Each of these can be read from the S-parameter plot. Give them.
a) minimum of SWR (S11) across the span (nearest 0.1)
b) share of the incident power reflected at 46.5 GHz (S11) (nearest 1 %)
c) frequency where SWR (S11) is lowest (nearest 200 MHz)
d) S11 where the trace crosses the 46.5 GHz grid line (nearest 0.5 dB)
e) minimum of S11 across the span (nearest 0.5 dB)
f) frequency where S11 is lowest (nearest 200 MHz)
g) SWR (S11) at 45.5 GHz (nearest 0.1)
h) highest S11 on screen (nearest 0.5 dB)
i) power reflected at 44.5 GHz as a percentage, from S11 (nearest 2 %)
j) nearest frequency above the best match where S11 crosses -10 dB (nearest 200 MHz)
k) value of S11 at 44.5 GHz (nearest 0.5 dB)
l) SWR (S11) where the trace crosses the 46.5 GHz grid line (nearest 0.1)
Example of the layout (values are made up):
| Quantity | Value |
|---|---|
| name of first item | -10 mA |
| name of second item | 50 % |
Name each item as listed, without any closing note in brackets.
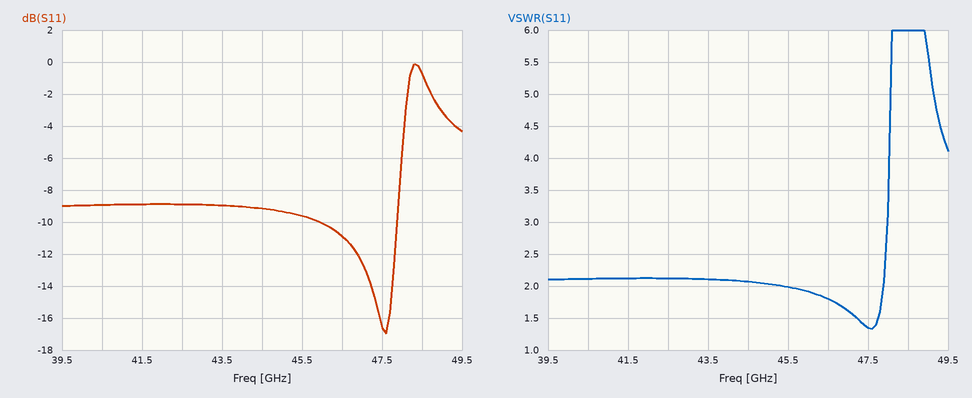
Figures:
| Quantity | Value |
|---|---|
| minimum of SWR (S11) across the span | 1.3 |
| share of the incident power reflected at 46.5 GHz (S11) | 8 % |
| frequency where SWR (S11) is lowest | 47.6 GHz |
| S11 where the trace crosses the 46.5 GHz grid line | -11.0 dB |
| minimum of S11 across the span | -17.0 dB |
| frequency where S11 is lowest | 47.6 GHz |
| SWR (S11) at 45.5 GHz | 2.0 |
| highest S11 on screen | 0.0 dB |
| power reflected at 44.5 GHz as a percentage, from S11 | 12 % |
| nearest frequency above the best match where S11 crosses -10 dB | 47.8 GHz |
| value of S11 at 44.5 GHz | -9.0 dB |
| SWR (S11) where the trace crosses the 46.5 GHz grid line | 1.8 |
